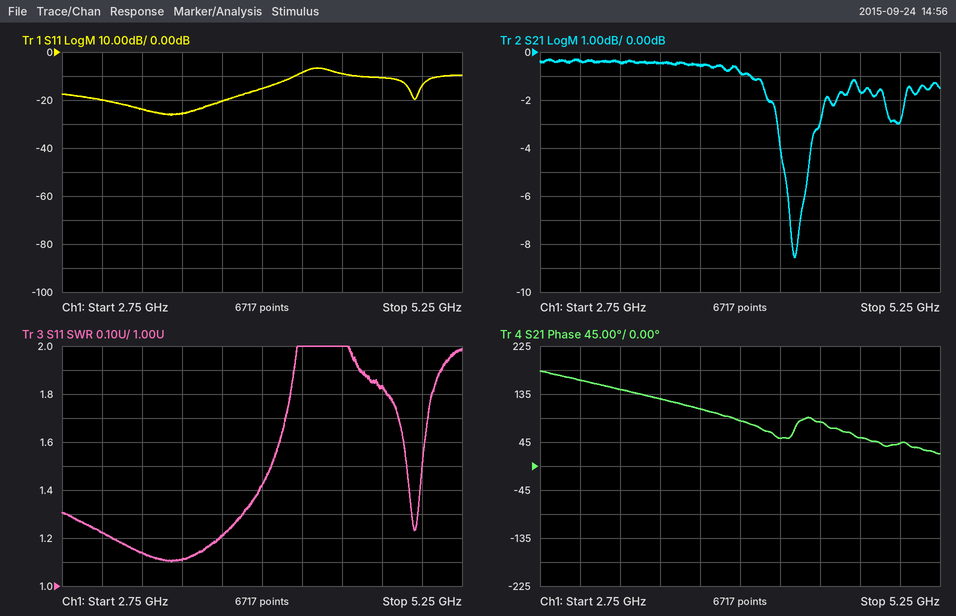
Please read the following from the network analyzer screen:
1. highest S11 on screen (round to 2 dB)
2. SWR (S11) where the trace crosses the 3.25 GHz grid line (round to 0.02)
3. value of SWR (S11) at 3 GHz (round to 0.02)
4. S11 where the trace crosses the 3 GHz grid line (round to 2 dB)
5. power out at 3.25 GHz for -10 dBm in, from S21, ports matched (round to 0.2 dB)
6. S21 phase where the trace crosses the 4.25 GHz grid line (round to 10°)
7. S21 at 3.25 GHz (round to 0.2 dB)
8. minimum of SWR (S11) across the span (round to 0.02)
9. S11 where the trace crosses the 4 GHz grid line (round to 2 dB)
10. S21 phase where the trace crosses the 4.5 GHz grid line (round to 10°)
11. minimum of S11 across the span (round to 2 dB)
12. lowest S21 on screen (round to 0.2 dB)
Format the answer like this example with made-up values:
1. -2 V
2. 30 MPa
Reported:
1. -6 dB
2. 1.14
3. 1.22
4. -20 dB
5. -10.4 dBm
6. 50°
7. -0.4 dB
8. 1.10
9. -16 dB
10. 80°
11. -26 dB
12. -8.6 dB
